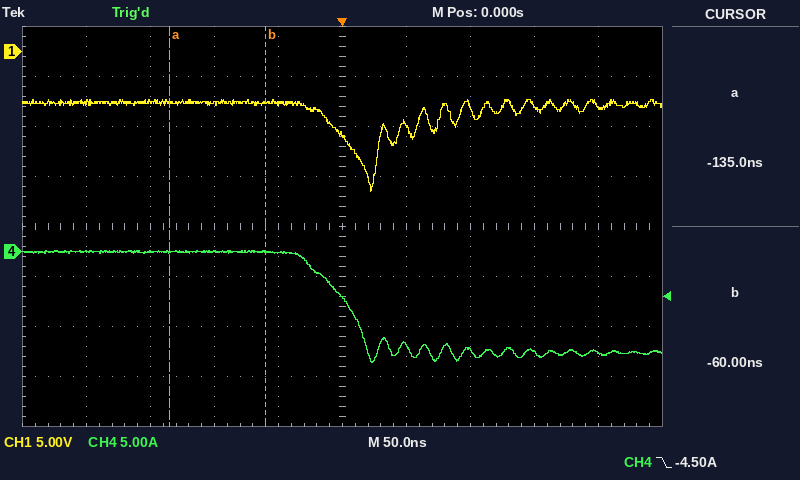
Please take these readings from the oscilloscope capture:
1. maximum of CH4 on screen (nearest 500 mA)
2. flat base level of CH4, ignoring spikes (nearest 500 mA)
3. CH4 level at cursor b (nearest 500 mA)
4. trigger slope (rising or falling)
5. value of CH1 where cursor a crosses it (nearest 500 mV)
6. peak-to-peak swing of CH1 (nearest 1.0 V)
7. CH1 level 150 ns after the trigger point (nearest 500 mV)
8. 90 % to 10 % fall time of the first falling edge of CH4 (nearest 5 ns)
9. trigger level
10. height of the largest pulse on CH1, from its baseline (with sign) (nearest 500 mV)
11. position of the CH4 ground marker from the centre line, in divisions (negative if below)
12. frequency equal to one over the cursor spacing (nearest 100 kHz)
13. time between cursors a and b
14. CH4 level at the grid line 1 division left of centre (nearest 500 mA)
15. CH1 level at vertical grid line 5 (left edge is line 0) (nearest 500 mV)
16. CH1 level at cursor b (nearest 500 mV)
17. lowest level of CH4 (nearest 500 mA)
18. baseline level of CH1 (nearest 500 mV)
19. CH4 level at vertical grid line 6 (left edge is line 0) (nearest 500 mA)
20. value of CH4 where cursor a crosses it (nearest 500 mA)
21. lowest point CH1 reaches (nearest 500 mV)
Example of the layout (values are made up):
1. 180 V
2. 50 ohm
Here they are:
1. 0.0 A
2. -10.0 A
3. 0.0 A
4. falling
5. -5.0 V
6. 9.0 V
7. -5.5 V
8. 45 ns
9. -4.50 A
10. -9.0 V
11. -0.5 div
12. 13.3 MHz
13. 75 ns
14. 0.0 A
15. -8.5 V
16. -5.0 V
17. -11.0 A
18. -5.0 V
19. -9.5 A
20. 0.0 A
21. -14.0 V
